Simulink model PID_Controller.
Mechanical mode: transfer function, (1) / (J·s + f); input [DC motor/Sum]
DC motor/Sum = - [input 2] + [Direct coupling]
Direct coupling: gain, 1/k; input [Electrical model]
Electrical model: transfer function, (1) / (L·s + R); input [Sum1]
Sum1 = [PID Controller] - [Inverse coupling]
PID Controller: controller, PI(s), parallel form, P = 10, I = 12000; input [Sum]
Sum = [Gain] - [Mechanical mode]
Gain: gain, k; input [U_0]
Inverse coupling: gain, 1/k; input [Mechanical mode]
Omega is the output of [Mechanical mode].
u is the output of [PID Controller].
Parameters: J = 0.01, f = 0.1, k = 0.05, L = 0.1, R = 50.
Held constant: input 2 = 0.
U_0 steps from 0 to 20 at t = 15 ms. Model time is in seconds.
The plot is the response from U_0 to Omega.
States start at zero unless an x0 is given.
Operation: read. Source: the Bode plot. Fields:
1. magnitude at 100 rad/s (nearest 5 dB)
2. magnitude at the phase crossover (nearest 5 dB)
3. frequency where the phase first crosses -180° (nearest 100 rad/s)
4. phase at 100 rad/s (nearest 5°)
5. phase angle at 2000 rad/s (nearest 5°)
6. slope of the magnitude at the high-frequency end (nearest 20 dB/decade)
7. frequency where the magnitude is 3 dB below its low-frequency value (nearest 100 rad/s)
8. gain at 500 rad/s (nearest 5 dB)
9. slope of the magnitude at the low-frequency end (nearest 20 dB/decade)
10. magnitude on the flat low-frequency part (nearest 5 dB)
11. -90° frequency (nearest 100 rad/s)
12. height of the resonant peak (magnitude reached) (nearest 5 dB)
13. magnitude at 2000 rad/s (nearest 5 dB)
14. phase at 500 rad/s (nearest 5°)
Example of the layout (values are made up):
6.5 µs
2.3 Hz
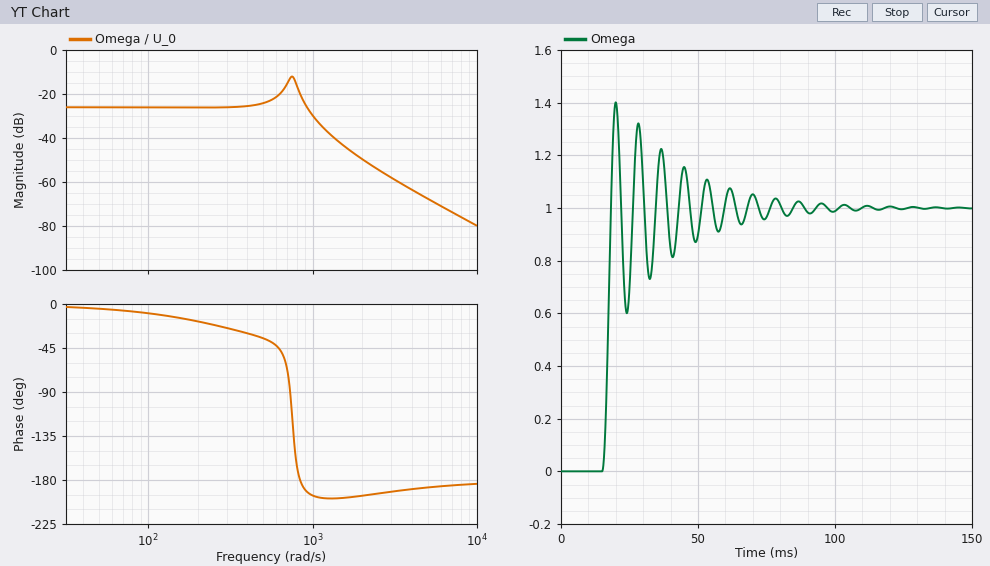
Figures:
-25 dB
-20 dB
800 rad/s
-10°
-195°
-40 dB/decade
1000 rad/s
-25 dB
0 dB/decade
-25 dB
700 rad/s
-10 dB
-50 dB
-35°
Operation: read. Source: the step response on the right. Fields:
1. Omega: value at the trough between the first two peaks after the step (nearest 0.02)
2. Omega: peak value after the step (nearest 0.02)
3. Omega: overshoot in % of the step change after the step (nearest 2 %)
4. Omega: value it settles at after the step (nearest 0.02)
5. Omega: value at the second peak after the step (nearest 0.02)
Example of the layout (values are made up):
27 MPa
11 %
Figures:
0.60
1.40
40 %
1.00
1.32
